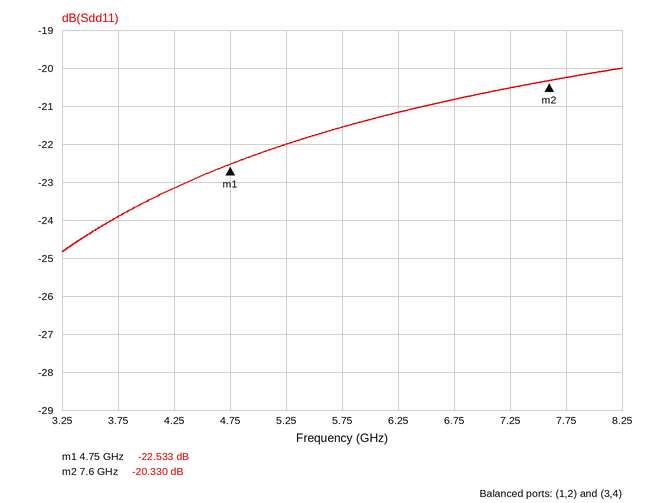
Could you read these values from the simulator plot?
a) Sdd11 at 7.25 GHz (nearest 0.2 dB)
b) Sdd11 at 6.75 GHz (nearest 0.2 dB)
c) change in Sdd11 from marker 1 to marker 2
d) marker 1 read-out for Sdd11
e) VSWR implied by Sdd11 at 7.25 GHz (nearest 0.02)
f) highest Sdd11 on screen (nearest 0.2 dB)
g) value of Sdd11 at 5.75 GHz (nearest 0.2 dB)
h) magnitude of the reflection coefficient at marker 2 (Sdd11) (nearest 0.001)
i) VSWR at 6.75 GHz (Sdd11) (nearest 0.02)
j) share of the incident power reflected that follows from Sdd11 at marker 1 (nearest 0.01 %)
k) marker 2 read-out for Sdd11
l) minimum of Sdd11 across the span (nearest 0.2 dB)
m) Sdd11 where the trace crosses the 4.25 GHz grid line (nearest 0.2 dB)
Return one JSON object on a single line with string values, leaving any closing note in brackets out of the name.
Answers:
{"Sdd11 at 7.25 GHz": "-20.6 dB", "Sdd11 at 6.75 GHz": "-20.8 dB", "change in Sdd11 from marker 1 to marker 2": "2.203 dB", "marker 1 read-out for Sdd11": "-22.533 dB", "VSWR implied by Sdd11 at 7.25 GHz": "1.20", "highest Sdd11 on screen": "-20.0 dB", "value of Sdd11 at 5.75 GHz": "-21.6 dB", "magnitude of the reflection coefficient at marker 2 (Sdd11)": "0.096", "VSWR at 6.75 GHz (Sdd11)": "1.20", "share of the incident power reflected that follows from Sdd11 at marker 1": "0.56 %", "marker 2 read-out for Sdd11": "-20.330 dB", "minimum of Sdd11 across the span": "-24.8 dB", "Sdd11 where the trace crosses the 4.25 GHz grid line": "-23.2 dB"}
